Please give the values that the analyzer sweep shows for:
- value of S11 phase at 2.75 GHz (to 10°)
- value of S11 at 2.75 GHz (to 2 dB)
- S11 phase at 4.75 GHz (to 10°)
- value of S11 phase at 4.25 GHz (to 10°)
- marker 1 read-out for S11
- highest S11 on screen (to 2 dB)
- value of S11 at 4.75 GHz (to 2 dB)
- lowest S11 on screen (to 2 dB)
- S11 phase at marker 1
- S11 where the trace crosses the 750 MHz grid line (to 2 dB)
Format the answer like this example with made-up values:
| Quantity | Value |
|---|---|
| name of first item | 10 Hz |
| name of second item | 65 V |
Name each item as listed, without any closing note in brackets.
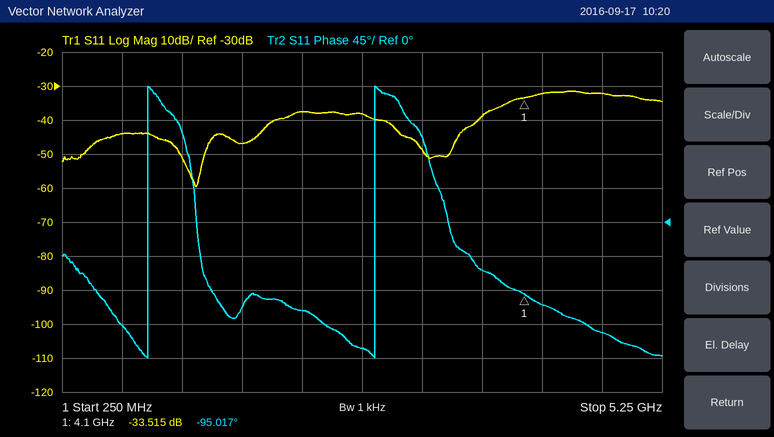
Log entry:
| Quantity | Value |
|---|---|
| value of S11 phase at 2.75 GHz | -170° |
| value of S11 at 2.75 GHz | -38 dB |
| S11 phase at 4.75 GHz | -150° |
| value of S11 phase at 4.25 GHz | -110° |
| marker 1 read-out for S11 | -33.515 dB |
| highest S11 on screen | -32 dB |
| value of S11 at 4.75 GHz | -32 dB |
| lowest S11 on screen | -60 dB |
| S11 phase at marker 1 | -95.017° |
| S11 where the trace crosses the 750 MHz grid line | -44 dB |
